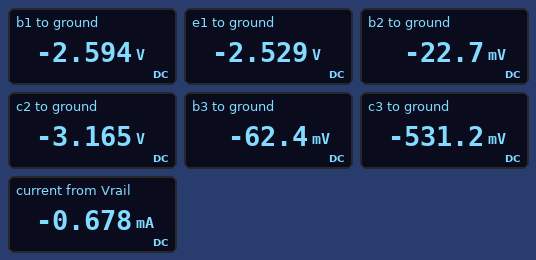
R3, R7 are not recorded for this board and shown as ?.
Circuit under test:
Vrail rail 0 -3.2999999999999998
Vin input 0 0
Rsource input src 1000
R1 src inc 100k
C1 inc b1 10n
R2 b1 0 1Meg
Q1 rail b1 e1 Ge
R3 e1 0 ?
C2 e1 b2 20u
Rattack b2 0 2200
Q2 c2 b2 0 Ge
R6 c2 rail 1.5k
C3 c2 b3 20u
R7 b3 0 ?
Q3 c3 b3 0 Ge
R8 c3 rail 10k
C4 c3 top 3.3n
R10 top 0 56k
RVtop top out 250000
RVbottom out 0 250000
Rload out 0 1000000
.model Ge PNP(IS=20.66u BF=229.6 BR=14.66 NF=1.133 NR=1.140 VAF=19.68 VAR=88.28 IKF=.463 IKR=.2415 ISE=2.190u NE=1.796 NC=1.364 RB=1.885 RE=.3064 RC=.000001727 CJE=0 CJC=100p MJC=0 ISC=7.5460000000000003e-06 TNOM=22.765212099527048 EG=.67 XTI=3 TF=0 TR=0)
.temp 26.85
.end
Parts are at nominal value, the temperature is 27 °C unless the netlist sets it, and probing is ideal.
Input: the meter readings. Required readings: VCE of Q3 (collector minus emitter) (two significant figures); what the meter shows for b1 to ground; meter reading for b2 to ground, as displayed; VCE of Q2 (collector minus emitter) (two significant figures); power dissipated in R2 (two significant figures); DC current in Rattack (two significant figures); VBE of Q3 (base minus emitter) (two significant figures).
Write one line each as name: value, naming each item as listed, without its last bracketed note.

VCE of Q3 (collector minus emitter): -530 mV
what the meter shows for b1 to ground: -2.594 V
meter reading for b2 to ground, as displayed: -22.7 mV
VCE of Q2 (collector minus emitter): -3.2 V
power dissipated in R2: 6.7 µW
DC current in Rattack: 10 µA
VBE of Q3 (base minus emitter): -62 mV
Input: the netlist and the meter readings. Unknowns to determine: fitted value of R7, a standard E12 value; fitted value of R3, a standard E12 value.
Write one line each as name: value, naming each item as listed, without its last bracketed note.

fitted value of R7, a standard E12 value: 18 kΩ
fitted value of R3, a standard E12 value: 8.2 kΩ
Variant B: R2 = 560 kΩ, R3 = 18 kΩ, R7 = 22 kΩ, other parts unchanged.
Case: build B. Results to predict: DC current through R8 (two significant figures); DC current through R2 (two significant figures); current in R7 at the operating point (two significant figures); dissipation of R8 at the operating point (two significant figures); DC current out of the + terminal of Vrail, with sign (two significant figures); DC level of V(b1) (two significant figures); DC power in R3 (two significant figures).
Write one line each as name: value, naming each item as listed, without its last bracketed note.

DC current through R8: 290 µA
DC current through R2: 5.7 µA
current in R7 at the operating point: 2.9 µA
dissipation of R8 at the operating point: 860 µW
DC current out of the + terminal of Vrail, with sign: -560 µA
DC level of V(b1): -3.2 V
DC power in R3: 550 µW
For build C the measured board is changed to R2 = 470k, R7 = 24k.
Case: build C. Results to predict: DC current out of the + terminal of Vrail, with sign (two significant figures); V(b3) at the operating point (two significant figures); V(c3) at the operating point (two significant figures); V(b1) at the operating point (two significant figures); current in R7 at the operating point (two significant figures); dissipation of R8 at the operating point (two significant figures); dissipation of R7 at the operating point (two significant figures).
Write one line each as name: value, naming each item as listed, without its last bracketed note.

DC current out of the + terminal of Vrail, with sign: -640 µA
V(b3) at the operating point: -65 mV
V(c3) at the operating point: -310 mV
V(b1) at the operating point: -2.1 V
current in R7 at the operating point: 2.7 µA
dissipation of R8 at the operating point: 890 µW
dissipation of R7 at the operating point: 180 nW
